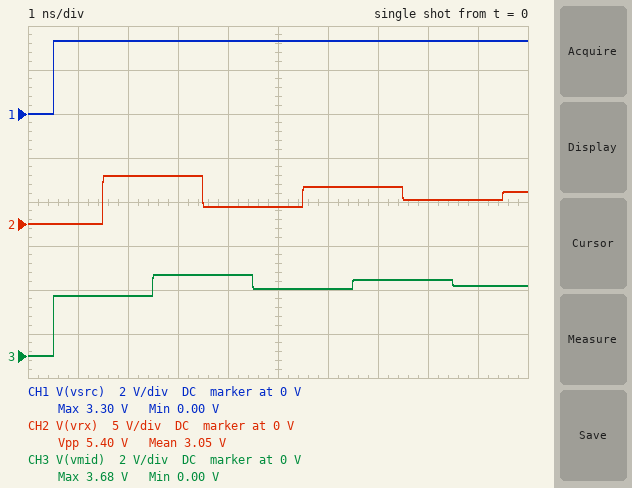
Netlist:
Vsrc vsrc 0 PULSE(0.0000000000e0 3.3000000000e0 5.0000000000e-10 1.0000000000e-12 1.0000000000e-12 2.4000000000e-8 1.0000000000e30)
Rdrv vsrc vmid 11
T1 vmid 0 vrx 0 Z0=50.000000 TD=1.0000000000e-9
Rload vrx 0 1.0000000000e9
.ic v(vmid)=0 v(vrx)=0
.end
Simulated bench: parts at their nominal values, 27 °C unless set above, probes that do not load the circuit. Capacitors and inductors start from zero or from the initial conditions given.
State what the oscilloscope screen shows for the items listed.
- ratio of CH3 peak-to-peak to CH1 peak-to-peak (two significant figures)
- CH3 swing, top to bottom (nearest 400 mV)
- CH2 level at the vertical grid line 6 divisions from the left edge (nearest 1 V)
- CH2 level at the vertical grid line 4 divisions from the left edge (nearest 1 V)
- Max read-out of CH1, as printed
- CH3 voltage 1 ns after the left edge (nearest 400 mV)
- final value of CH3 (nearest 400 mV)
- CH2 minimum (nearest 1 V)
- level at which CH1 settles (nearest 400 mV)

1.1
3.6 V
4 V
2 V
3.30 V
2.8 V
3.2 V
0 V
3.2 V
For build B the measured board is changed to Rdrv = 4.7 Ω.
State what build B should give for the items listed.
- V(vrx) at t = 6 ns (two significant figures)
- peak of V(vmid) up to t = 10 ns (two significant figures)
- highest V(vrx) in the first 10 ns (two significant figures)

5.2 V
3.5 V
6.0 V
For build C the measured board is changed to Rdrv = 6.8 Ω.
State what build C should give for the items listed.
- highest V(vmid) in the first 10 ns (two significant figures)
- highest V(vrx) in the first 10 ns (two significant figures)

3.6 V
5.8 V
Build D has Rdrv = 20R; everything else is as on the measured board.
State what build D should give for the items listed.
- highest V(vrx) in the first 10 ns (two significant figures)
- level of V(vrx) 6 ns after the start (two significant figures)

4.7 V
3.6 V
